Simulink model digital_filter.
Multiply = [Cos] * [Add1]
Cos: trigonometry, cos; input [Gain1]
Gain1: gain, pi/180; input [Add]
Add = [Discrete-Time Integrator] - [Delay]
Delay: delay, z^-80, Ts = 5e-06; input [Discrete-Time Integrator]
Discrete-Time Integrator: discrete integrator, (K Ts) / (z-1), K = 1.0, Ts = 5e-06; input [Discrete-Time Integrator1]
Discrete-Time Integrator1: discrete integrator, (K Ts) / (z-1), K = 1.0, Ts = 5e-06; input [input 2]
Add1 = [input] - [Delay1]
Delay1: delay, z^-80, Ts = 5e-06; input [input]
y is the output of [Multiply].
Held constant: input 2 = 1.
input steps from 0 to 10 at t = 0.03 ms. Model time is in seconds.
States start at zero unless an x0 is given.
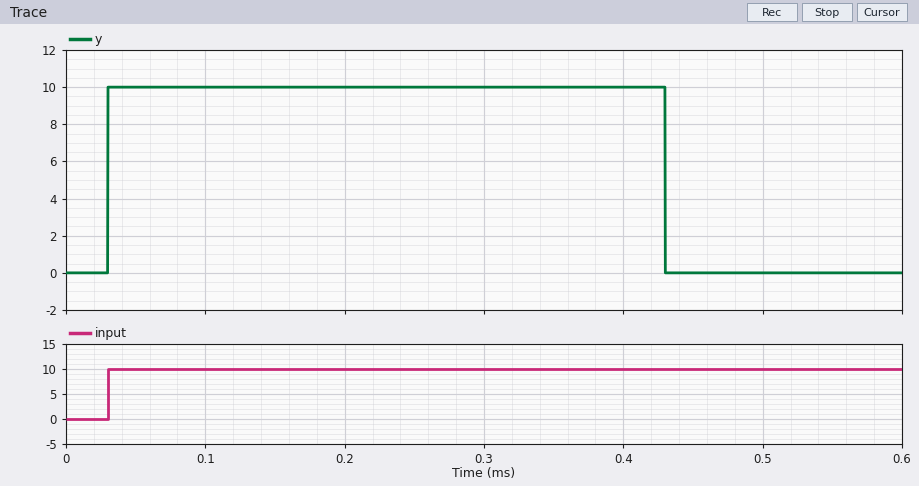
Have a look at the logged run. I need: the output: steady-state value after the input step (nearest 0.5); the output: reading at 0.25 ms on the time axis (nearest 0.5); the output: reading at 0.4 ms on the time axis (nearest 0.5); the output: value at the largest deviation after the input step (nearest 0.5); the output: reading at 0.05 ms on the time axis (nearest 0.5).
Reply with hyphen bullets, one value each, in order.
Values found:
- 0.0
- 10.0
- 10.0
- 10.0
- 10.0
